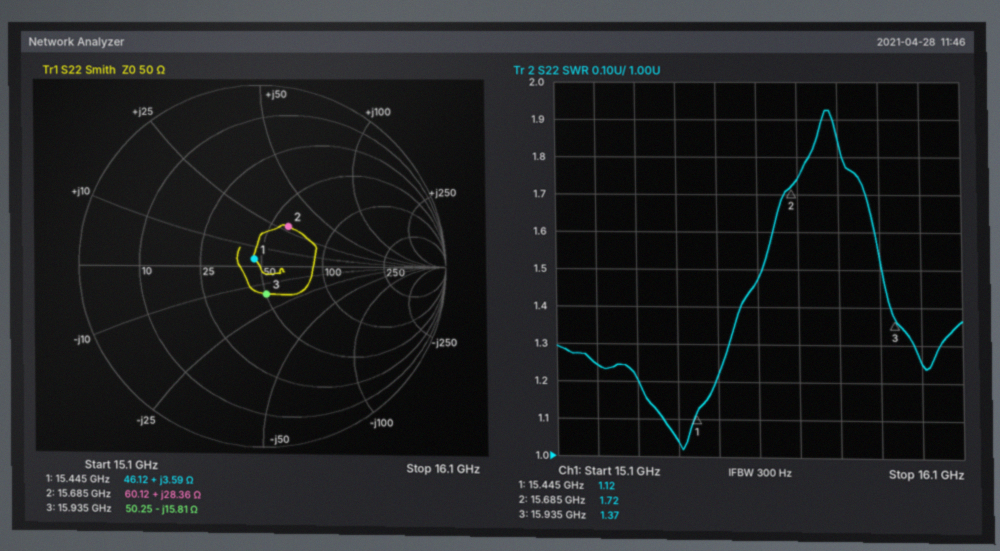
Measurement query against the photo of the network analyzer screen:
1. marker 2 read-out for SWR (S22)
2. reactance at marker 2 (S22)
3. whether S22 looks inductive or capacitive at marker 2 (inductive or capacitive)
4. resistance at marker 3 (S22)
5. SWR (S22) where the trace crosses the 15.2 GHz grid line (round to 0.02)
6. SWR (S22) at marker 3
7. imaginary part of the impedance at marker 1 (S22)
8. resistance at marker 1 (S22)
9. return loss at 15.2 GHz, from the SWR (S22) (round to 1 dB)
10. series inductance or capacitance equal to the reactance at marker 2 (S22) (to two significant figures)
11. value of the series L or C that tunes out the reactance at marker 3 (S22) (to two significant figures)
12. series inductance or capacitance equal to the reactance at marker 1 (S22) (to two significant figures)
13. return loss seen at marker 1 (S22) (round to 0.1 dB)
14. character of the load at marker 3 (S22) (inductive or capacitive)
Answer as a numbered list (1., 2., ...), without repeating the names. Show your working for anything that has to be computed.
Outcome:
1. 1.72
2. +28.36 Ω
3. inductive
4. 50.25 Ω
5. 1.24
6. 1.37
7. +3.59 Ω
8. 46.12 Ω
9. −20 log10((1.24 − 1)/(1.24 + 1)) ≈ 19 dB
10. L = 28.36 Ω/(2π × 15.685 GHz) ≈ 288 pH, so 290 pH to two significant figures
11. L = 15.81 Ω/(2π × 15.935 GHz) ≈ 158 pH, so 160 pH to two significant figures
12. L = 3.59 Ω/(2π × 15.445 GHz) ≈ 37 pH
13. 25.2 dB
14. capacitive
